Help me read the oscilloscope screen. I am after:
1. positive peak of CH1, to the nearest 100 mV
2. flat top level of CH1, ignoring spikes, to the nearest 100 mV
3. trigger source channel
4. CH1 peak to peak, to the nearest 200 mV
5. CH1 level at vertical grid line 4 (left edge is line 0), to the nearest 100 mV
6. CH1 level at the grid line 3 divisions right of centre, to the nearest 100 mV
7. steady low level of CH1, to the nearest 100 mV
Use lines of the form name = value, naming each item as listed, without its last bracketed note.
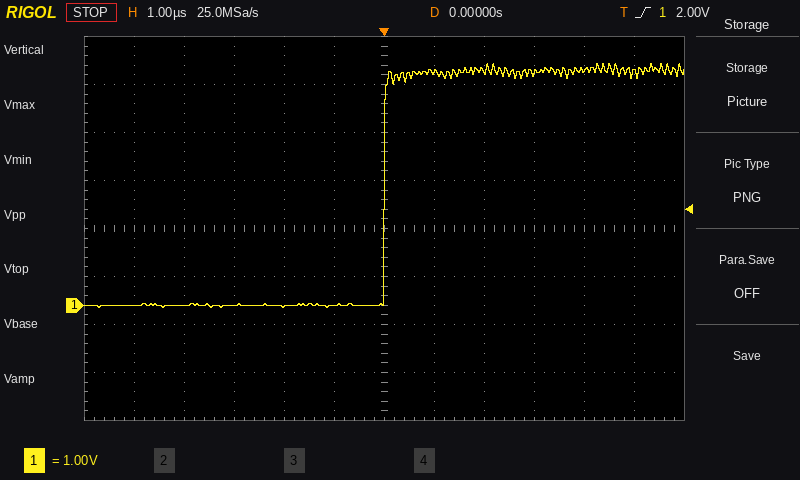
positive peak of CH1, to the nearest 100 mV = 5.0 V
flat top level of CH1, ignoring spikes, to the nearest 100 mV = 4.9 V
trigger source channel = CH1
CH1 peak to peak, to the nearest 200 mV = 5.0 V
CH1 level at vertical grid line 4 (left edge is line 0), to the nearest 100 mV = 0.0 V
CH1 level at the grid line 3 divisions right of centre, to the nearest 100 mV = 4.8 V
steady low level of CH1, to the nearest 100 mV = 0.0 V
